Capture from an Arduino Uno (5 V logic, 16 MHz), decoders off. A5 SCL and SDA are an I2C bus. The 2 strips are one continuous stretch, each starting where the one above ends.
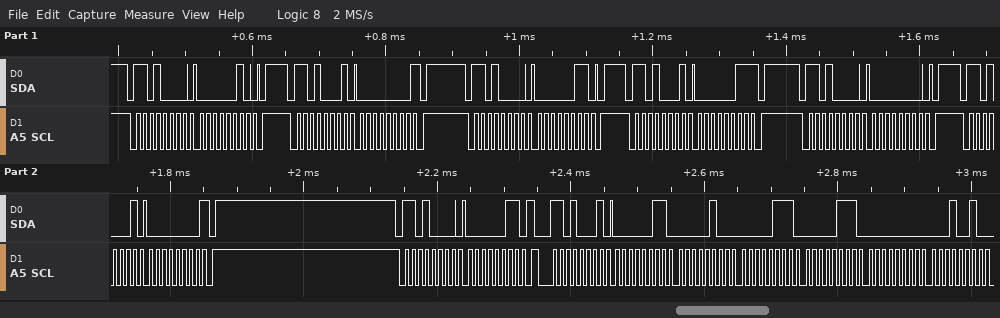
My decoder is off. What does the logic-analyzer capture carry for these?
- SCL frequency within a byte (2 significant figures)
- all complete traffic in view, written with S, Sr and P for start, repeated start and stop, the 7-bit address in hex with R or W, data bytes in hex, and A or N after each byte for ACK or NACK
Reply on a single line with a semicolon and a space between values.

100 kHz; S 68W A 02 A P S 68R A 00 N P S 68W A 03 A P S 68R A 03 N P S 68W A 00 A P S 68R A 00 N P S 68W A 03 A Sr 68R A 03 A 04 A 07 A 07 A 00 A 12 A
